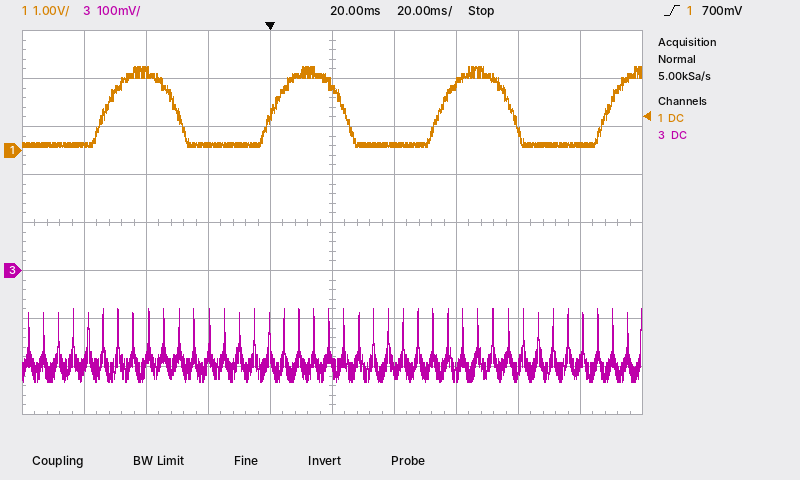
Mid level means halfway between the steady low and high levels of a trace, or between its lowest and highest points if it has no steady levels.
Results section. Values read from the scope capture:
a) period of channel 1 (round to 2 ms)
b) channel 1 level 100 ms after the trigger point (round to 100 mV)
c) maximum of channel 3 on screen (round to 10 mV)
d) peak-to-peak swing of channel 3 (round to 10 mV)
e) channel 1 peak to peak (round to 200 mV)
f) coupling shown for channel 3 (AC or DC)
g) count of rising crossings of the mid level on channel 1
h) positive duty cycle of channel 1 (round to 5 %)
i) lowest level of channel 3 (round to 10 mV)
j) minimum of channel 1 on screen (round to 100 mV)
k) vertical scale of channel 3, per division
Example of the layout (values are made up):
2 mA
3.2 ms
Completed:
54 ms
100 mV
-80 mV
150 mV
1.6 V
DC
4
40 %
-230 mV
100 mV
100 mV
